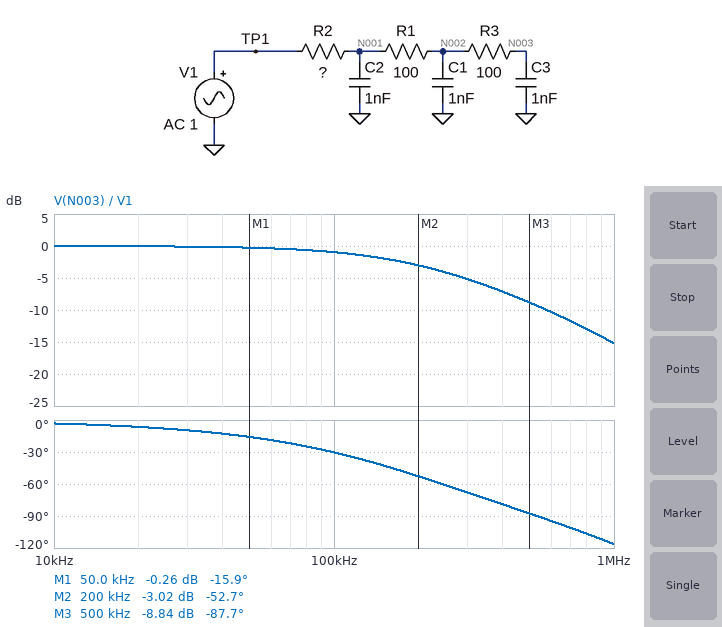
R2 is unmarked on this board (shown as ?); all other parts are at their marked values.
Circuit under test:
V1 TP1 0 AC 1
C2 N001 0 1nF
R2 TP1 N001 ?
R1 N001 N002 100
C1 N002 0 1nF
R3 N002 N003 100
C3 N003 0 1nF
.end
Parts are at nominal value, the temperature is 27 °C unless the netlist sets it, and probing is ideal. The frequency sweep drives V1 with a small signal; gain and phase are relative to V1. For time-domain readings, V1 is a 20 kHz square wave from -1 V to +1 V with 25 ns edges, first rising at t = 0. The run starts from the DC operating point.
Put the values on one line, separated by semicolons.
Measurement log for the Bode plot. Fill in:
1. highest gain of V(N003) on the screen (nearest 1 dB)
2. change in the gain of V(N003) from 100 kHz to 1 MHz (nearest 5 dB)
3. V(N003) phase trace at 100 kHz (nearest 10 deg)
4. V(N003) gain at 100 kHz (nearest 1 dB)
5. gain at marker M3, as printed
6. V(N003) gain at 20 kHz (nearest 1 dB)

0 dB; -15 dB; -30 deg; -1 dB; -8.84 dB; 0 dB
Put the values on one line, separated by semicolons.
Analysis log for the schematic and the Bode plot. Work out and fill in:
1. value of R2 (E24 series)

200 Ω
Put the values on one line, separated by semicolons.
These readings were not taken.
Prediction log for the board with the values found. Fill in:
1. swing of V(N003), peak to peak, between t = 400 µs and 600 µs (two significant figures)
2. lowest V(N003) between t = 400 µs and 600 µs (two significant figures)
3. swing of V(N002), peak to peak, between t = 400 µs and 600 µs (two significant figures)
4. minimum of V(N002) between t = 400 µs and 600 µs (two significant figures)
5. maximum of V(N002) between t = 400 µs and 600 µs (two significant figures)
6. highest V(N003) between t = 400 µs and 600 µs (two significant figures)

2.0 V; -1.0 V; 2.0 V; -1.0 V; 1.0 V; 1.0 V
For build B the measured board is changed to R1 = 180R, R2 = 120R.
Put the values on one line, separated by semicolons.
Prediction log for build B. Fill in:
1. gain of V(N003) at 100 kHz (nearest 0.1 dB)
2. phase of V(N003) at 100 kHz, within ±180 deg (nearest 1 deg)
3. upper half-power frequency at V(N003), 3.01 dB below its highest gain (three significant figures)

-0.8 dB; -28 deg; 223 kHz
